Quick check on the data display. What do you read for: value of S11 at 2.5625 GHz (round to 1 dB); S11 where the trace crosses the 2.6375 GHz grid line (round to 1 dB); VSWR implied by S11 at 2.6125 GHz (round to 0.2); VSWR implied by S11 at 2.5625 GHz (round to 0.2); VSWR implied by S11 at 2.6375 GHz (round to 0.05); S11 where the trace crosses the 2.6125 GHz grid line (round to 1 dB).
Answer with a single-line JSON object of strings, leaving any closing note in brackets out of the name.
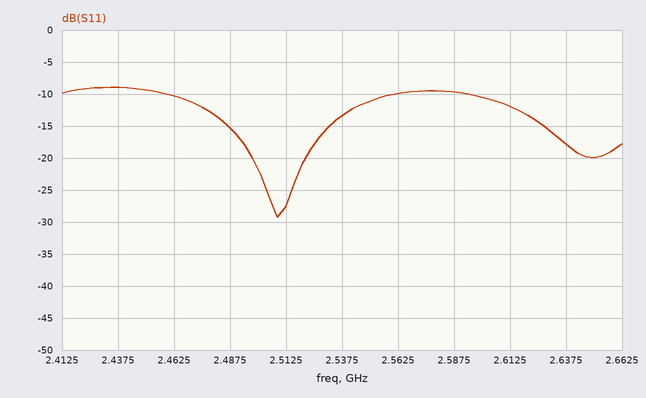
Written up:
{"value of S11 at 2.5625 GHz": "-10 dB", "S11 where the trace crosses the 2.6375 GHz grid line": "-18 dB", "VSWR implied by S11 at 2.6125 GHz": "1.6", "VSWR implied by S11 at 2.5625 GHz": "2.0", "VSWR implied by S11 at 2.6375 GHz": "1.30", "S11 where the trace crosses the 2.6125 GHz grid line": "-12 dB"}
